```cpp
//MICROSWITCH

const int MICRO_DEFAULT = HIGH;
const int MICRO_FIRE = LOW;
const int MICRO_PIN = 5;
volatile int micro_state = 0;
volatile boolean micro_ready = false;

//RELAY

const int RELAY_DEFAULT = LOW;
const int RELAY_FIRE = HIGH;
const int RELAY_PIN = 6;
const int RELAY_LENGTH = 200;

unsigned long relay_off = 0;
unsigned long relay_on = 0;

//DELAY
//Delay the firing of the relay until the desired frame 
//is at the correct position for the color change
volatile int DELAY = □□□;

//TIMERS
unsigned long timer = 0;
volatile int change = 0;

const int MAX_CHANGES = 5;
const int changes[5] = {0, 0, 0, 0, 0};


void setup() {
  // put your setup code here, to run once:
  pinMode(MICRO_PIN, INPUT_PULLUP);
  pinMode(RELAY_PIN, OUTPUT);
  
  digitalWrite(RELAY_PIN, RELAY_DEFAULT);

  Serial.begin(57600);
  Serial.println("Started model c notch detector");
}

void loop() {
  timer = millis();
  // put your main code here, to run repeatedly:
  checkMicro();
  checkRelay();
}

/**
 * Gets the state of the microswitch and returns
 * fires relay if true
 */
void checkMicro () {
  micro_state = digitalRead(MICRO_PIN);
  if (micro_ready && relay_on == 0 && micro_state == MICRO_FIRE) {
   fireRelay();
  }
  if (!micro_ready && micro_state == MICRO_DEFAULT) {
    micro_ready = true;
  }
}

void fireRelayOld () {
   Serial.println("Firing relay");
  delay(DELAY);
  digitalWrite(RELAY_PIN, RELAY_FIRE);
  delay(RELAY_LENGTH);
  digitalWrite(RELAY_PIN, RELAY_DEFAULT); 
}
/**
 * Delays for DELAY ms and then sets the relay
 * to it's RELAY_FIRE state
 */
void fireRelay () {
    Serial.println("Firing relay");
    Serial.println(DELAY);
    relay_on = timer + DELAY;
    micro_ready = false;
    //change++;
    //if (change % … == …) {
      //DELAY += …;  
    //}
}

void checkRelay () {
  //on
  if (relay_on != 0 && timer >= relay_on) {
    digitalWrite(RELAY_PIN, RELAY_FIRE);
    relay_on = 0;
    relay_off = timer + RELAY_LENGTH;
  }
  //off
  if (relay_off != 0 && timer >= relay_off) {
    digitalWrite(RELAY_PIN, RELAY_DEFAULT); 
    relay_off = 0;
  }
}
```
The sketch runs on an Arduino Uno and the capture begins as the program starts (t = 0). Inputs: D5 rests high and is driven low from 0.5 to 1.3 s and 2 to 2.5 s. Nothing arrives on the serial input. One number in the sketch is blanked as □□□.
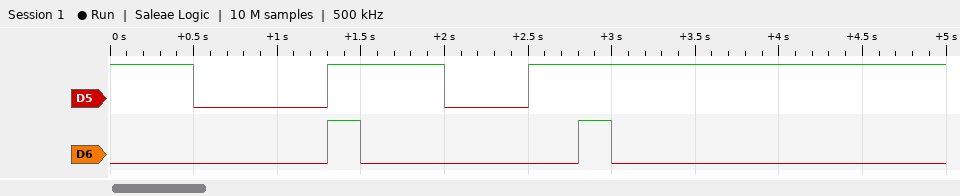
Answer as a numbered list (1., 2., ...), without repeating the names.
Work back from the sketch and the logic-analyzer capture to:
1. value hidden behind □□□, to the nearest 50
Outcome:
1. 800
